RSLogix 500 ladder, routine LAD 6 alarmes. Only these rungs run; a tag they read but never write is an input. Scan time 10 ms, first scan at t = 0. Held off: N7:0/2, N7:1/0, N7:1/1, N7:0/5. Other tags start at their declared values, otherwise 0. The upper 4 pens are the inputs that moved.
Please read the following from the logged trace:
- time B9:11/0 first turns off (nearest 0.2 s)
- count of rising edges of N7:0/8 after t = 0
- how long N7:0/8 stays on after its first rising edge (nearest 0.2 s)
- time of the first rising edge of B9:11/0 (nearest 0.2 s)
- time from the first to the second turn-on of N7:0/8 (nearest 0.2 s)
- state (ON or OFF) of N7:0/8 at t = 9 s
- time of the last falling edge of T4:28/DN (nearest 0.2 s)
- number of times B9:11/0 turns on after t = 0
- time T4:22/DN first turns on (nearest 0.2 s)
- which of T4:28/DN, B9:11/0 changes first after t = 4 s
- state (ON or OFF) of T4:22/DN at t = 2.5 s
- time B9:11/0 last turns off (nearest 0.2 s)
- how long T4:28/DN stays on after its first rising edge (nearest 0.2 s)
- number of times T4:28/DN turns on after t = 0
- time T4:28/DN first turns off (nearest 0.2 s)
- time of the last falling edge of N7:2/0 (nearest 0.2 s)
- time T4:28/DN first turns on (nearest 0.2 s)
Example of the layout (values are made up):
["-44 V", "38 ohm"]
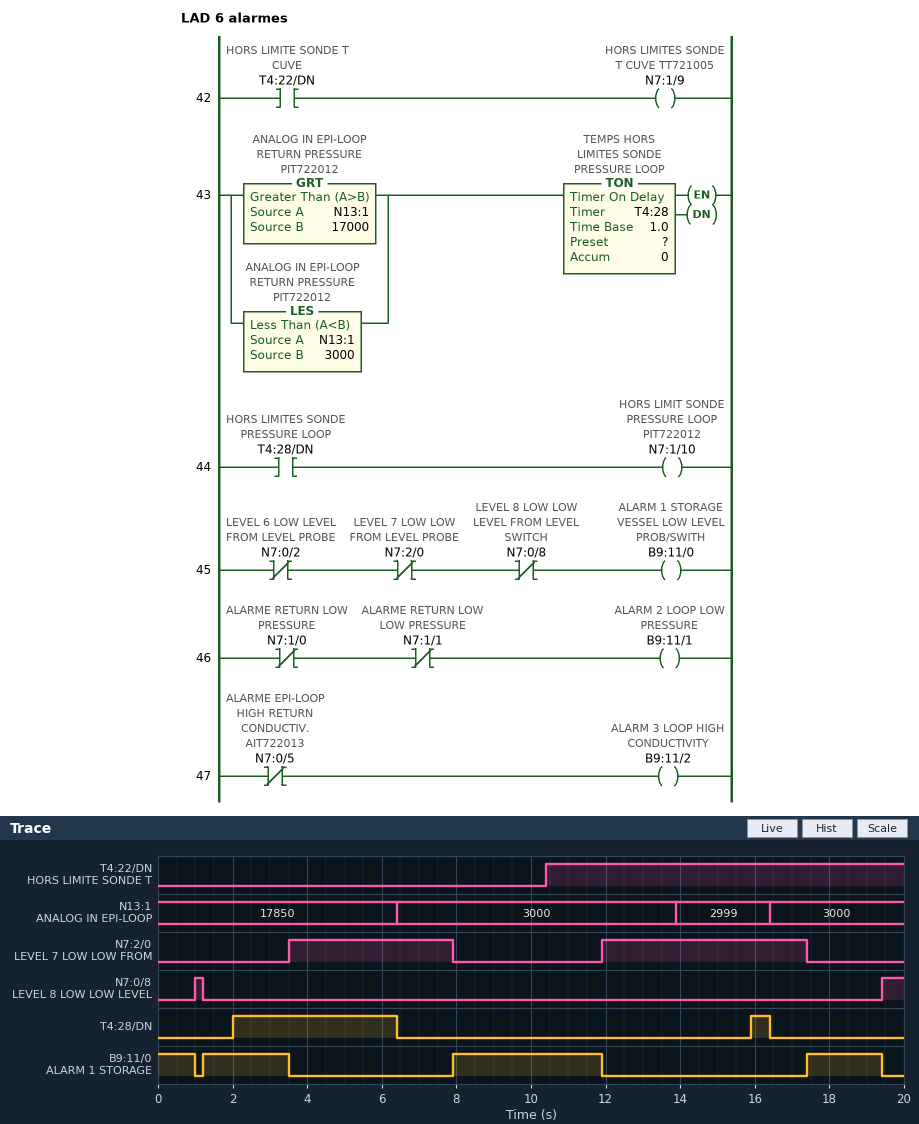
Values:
["1.0 s", "2", "0.2 s", "1.2 s", "18.4 s", "OFF", "16.4 s", "3", "10.4 s", "T4:28/DN", "OFF", "19.4 s", "4.4 s", "2", "6.4 s", "17.4 s", "2.0 s"]
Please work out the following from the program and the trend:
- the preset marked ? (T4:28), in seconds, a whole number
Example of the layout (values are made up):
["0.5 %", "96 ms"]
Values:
["2 s"]
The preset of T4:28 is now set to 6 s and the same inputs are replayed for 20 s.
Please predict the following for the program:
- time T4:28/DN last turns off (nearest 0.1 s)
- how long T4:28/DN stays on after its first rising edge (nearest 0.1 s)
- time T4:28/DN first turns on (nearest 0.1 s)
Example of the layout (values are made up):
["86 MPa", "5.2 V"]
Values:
["6.4 s", "0.4 s", "6.0 s"]
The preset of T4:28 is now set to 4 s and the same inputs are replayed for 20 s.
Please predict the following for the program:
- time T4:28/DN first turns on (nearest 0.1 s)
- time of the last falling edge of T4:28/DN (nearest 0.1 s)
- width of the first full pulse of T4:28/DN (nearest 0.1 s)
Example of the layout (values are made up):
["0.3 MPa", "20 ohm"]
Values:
["4.0 s", "6.4 s", "2.4 s"]
